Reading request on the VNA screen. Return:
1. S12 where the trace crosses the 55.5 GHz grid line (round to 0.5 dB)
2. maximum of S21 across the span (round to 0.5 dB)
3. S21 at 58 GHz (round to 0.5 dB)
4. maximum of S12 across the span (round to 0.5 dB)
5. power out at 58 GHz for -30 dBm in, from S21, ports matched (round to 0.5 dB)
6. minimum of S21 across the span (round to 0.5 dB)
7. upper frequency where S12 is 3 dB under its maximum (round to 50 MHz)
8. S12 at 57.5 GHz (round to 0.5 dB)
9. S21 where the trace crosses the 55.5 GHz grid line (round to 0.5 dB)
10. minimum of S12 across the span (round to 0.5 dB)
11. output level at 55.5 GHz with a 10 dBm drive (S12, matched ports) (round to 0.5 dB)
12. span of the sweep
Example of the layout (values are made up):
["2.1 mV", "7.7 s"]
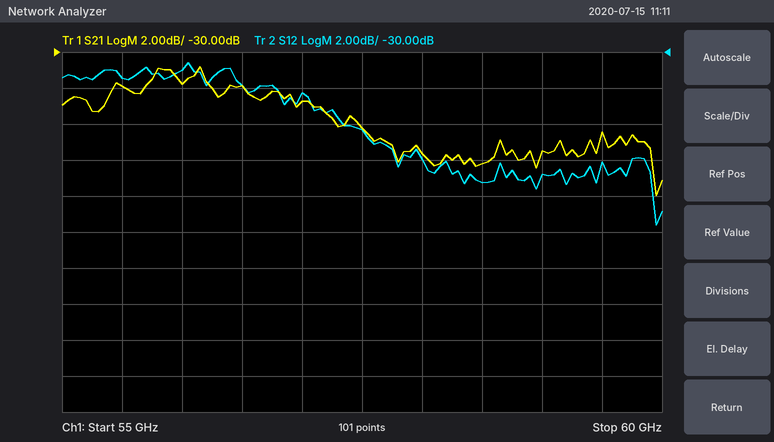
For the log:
["-31.5 dB", "-31.0 dB", "-35.5 dB", "-30.5 dB", "-65.5 dBm", "-38.0 dB", "57.30 GHz", "-34.5 dB", "-32.0 dB", "-39.5 dB", "-21.5 dBm", "5 GHz"]
